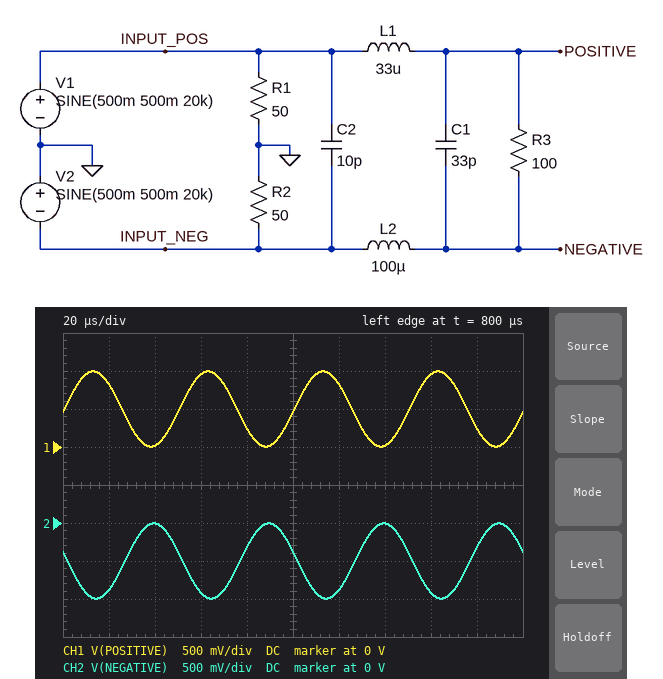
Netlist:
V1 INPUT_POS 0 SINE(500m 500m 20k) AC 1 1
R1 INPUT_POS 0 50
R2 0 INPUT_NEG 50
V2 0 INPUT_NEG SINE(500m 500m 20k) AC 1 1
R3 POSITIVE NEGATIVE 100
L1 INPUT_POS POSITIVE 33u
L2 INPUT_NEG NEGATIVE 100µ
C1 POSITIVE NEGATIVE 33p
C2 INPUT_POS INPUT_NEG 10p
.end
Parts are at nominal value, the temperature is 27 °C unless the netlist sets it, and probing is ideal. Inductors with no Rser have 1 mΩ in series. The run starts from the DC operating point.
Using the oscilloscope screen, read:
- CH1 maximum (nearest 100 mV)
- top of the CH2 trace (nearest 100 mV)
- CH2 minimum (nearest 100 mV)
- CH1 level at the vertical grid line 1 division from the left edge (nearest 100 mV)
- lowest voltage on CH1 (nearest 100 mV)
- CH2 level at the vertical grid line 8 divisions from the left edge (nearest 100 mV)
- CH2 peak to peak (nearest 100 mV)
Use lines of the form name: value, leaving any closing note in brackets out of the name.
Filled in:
CH1 maximum: 1.0 V
top of the CH2 trace: 0 V
CH2 minimum: -1.0 V
CH1 level at the vertical grid line 1 division from the left edge: 800 mV
lowest voltage on CH1: 0 V
CH2 level at the vertical grid line 8 divisions from the left edge: -900 mV
CH2 peak to peak: 1.0 V
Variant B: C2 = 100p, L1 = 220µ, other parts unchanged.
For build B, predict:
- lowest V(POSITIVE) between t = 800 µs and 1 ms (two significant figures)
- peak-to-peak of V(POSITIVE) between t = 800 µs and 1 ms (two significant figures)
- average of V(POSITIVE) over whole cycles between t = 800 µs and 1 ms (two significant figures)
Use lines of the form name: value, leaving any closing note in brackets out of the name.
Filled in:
lowest V(POSITIVE) between t = 800 µs and 1 ms: 31 mV
peak-to-peak of V(POSITIVE) between t = 800 µs and 1 ms: 940 mV
average of V(POSITIVE) over whole cycles between t = 800 µs and 1 ms: 500 mV
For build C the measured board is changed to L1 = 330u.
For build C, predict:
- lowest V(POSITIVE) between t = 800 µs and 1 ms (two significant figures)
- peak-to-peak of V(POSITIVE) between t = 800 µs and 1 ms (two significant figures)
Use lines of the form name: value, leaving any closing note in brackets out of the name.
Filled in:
lowest V(POSITIVE) between t = 800 µs and 1 ms: 42 mV
peak-to-peak of V(POSITIVE) between t = 800 µs and 1 ms: 920 mV
